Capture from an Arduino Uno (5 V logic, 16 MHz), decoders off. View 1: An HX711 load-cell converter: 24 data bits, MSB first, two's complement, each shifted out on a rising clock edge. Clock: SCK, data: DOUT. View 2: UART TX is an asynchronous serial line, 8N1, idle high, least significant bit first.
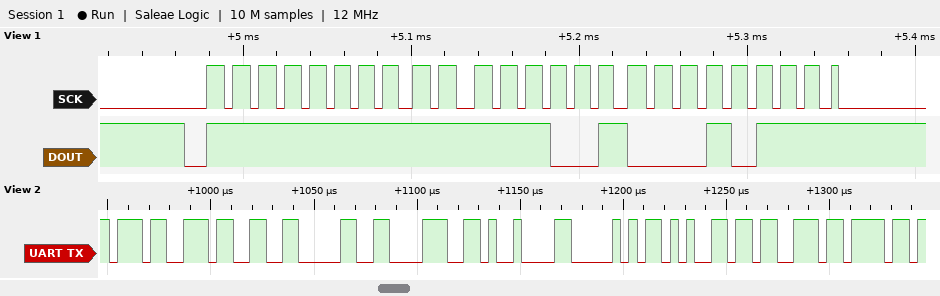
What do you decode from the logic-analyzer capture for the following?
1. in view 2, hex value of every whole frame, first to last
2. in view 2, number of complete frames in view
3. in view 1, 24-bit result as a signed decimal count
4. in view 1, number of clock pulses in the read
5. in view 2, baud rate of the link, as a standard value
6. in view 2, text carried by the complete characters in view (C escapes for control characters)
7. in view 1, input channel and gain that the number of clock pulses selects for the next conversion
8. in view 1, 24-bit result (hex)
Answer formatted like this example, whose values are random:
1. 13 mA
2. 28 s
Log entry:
1. 37 33 30 38 09 50 65 73 6F
2. 9
3. -1769
4. 25
5. 250000 baud
6. "7308\tPeso"
7. channel A, gain 128
8. 0xFFF917
